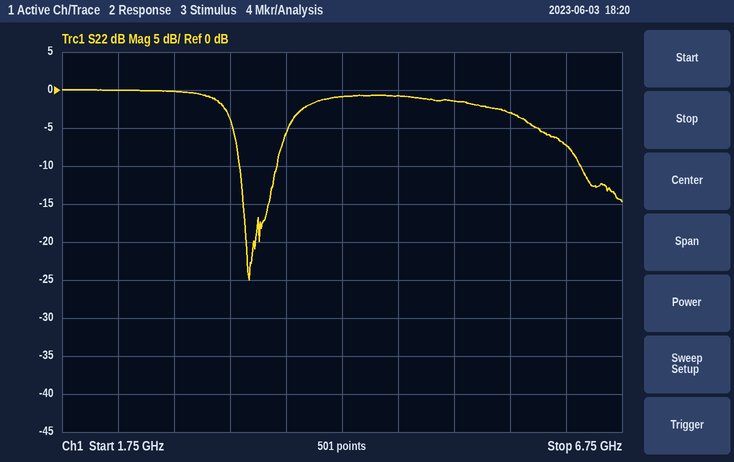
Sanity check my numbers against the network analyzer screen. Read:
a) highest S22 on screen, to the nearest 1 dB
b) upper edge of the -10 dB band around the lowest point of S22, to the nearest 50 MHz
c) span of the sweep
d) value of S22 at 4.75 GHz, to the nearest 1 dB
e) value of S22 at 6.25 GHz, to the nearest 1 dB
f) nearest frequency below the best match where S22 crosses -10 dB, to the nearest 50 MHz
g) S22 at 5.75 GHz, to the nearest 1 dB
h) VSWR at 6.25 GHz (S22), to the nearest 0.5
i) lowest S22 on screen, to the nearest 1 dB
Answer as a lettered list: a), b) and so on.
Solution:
a) 0 dB
b) 3.65 GHz
c) 5 GHz
d) -1 dB
e) -7 dB
f) 3.35 GHz
g) -3 dB
h) 2.5
i) -25 dB
